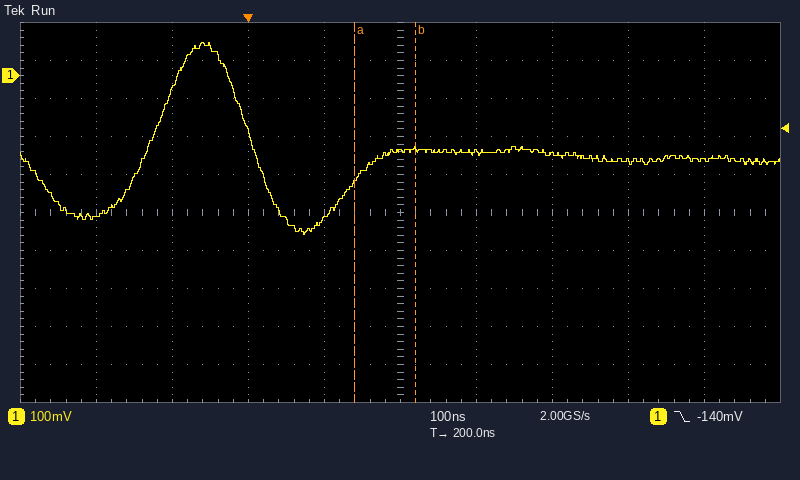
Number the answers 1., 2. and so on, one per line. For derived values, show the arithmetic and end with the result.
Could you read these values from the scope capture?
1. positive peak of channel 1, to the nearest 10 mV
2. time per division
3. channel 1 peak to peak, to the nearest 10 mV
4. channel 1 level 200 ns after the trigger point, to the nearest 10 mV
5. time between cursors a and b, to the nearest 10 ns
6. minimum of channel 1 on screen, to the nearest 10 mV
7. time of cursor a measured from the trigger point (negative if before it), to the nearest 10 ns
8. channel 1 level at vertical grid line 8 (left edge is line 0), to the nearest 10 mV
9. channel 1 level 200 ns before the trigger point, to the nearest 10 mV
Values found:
1. 90 mV
2. 100 ns
3. 90 mV − (-420 mV) = 510 mV
4. -200 mV
5. 80 ns
6. -420 mV
7. +140 ns
8. -230 mV
9. -370 mV
